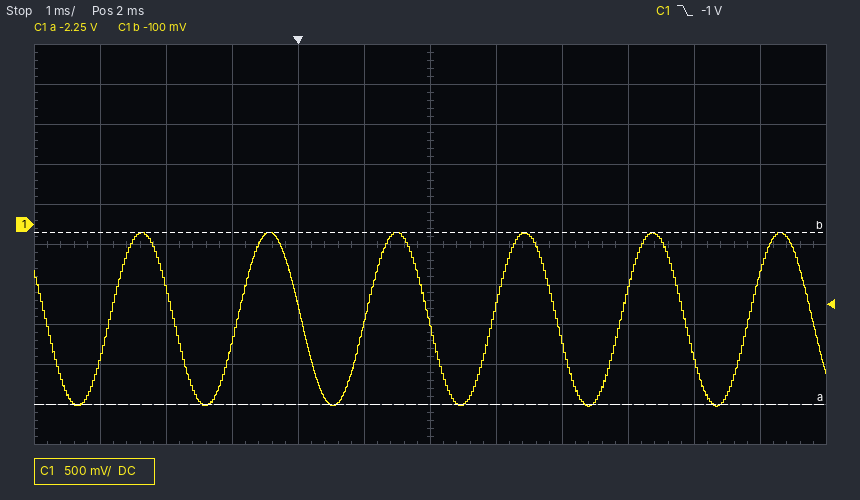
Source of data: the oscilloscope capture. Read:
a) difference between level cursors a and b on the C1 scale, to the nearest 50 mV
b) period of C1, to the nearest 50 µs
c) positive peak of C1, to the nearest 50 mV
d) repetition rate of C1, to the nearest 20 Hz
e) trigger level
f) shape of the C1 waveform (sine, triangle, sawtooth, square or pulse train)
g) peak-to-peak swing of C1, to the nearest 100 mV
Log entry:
2.15 V
1.95 ms
-100 mV
520 Hz
-1 V
sine
2.20 V
